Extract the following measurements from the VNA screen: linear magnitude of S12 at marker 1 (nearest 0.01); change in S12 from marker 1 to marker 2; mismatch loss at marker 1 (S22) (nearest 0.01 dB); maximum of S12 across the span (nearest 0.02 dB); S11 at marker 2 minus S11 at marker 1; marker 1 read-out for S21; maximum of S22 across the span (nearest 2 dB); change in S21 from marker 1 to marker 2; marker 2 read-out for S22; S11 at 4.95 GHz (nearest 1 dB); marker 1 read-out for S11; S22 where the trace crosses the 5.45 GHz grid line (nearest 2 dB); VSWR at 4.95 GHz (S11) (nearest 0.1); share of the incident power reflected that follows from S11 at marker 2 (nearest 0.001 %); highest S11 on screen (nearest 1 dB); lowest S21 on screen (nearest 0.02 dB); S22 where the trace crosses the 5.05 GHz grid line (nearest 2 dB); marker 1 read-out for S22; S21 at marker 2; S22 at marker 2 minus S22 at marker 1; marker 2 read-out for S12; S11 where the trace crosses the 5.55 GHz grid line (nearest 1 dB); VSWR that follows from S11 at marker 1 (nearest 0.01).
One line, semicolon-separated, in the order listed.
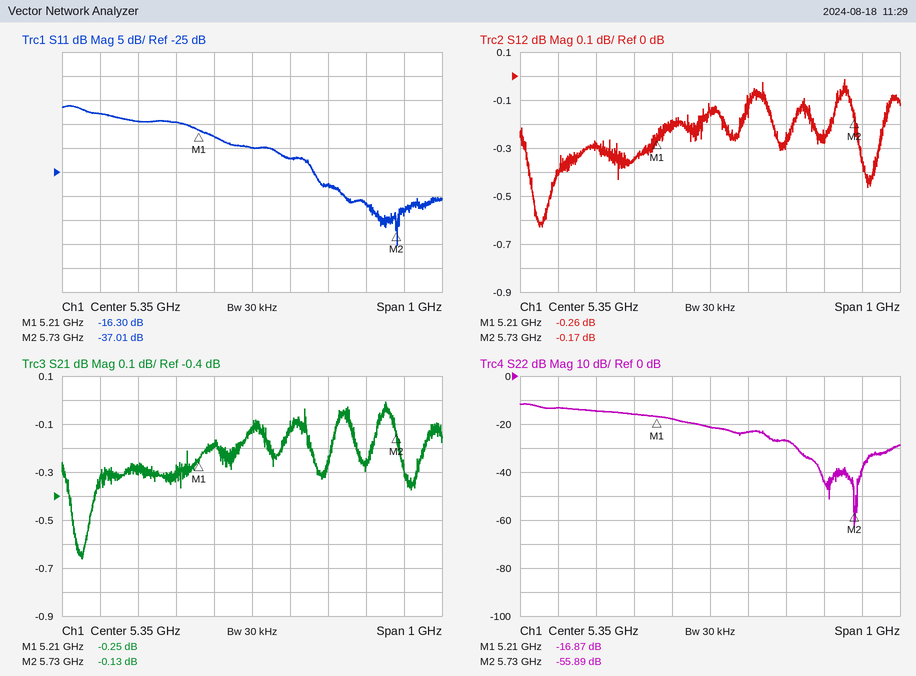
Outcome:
0.97; 0.09 dB; 0.09 dB; -0.02 dB; -20.71 dB; -0.25 dB; -12 dB; 0.12 dB; -55.89 dB; -13 dB; -16.30 dB; -24 dB; 1.6; 0.020 %; -11 dB; -0.66 dB; -14 dB; -16.87 dB; -0.13 dB; -39.02 dB; -0.17 dB; -28 dB; 1.36
